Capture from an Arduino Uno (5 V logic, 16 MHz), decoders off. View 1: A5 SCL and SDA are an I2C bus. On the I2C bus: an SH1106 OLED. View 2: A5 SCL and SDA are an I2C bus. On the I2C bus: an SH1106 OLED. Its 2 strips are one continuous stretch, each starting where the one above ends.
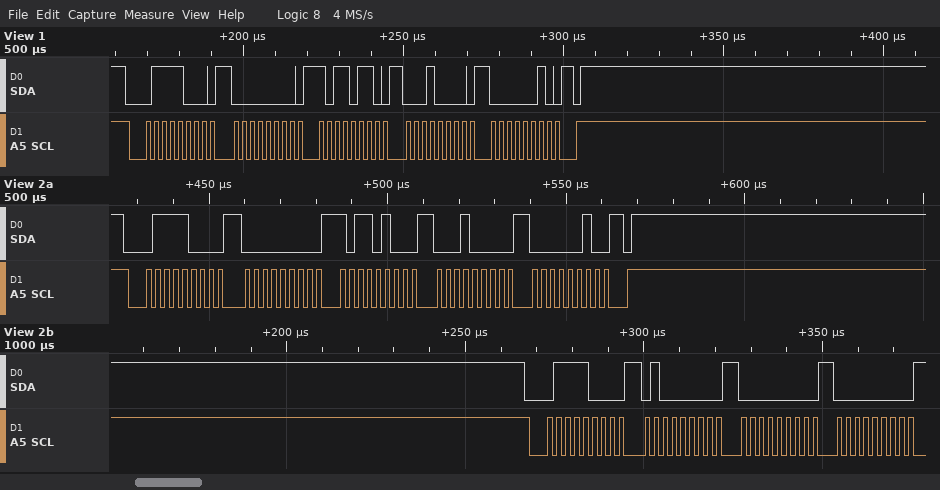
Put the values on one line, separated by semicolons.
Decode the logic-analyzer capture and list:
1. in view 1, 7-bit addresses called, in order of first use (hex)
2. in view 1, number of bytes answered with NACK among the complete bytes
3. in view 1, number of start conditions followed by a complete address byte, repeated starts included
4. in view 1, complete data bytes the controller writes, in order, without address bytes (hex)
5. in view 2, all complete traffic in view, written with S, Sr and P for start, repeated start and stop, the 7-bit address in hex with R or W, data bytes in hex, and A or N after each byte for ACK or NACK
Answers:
0x3C; 0; 1; 00 B6 10 02; S 3CW A 00 A B4 A 10 A 02 A P S 3CW A 40 A 00 A 00 A
